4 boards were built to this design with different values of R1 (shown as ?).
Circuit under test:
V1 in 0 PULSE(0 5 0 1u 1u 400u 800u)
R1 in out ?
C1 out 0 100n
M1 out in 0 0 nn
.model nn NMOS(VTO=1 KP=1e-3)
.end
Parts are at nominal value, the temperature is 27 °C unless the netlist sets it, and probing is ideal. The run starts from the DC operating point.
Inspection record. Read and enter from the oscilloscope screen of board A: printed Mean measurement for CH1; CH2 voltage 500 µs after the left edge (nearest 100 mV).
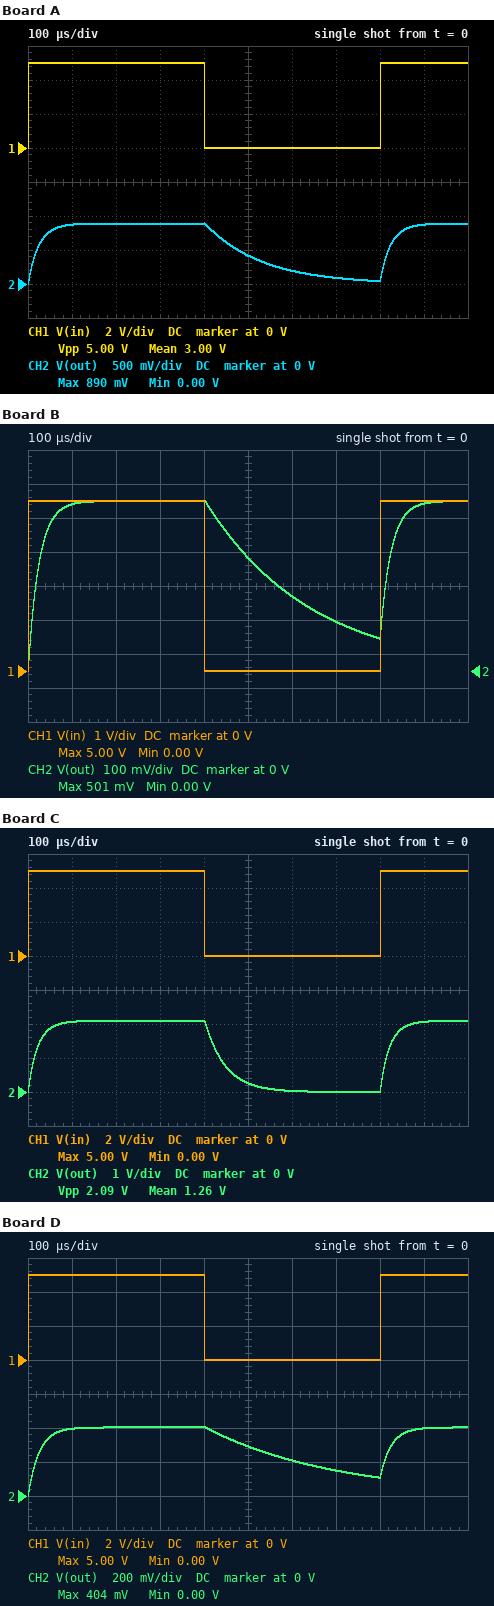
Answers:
3.00 V
400 mV
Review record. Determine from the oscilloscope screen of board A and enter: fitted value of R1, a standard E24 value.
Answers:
1.3 kΩ
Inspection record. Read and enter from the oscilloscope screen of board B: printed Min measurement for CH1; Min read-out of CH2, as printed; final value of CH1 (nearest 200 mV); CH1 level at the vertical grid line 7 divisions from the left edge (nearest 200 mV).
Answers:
0.00 V
0.00 V
5.0 V
0 V
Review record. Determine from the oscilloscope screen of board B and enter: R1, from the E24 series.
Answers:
2.4 kΩ
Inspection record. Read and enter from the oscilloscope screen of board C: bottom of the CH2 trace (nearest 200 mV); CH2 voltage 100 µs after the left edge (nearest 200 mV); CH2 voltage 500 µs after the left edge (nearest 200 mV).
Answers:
0 V
2.0 V
200 mV
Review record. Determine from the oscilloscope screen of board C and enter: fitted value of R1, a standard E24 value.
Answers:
470 Ω
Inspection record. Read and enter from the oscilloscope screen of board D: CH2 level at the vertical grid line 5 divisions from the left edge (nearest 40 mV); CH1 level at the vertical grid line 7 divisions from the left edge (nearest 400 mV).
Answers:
280 mV
0 V
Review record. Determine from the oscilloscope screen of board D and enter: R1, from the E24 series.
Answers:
3 kΩ
